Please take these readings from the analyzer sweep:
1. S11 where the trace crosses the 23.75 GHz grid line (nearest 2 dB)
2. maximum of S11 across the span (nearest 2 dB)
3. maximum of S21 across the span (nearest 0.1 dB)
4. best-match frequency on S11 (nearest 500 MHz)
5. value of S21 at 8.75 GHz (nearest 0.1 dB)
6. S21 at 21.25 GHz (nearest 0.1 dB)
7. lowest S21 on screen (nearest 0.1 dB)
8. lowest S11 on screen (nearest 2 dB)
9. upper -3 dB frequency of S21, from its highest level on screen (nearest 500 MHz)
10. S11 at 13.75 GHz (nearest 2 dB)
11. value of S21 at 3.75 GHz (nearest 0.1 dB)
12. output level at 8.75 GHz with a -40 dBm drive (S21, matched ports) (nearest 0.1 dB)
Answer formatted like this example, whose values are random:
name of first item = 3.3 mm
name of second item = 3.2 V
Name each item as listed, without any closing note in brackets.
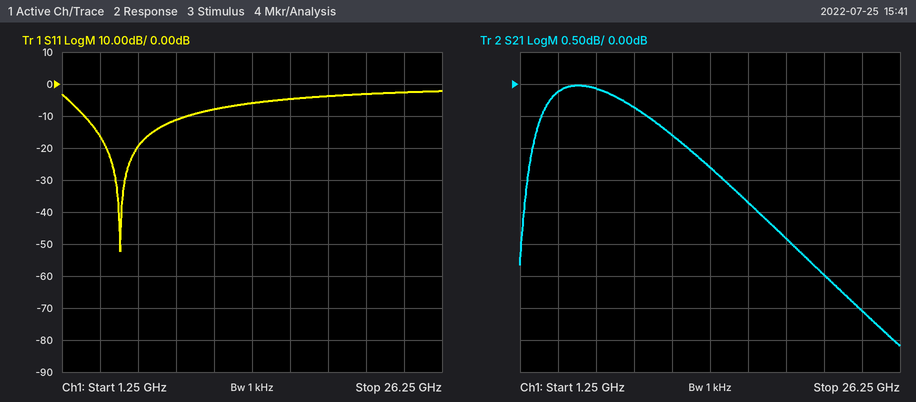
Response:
S11 where the trace crosses the 23.75 GHz grid line = -2 dB
maximum of S11 across the span = -2 dB
maximum of S21 across the span = 0.0 dB
best-match frequency on S11 = 5.0 GHz
value of S21 at 8.75 GHz = -0.4 dB
S21 at 21.25 GHz = -3.0 dB
lowest S21 on screen = -4.1 dB
lowest S11 on screen = -52 dB
upper -3 dB frequency of S21, from its highest level on screen = 21.5 GHz
S11 at 13.75 GHz = -6 dB
value of S21 at 3.75 GHz = -0.1 dB
output level at 8.75 GHz with a -40 dBm drive (S21, matched ports) = -40.4 dBm
